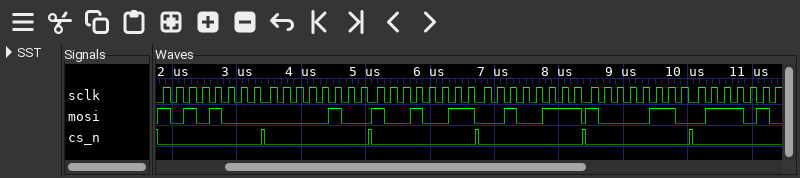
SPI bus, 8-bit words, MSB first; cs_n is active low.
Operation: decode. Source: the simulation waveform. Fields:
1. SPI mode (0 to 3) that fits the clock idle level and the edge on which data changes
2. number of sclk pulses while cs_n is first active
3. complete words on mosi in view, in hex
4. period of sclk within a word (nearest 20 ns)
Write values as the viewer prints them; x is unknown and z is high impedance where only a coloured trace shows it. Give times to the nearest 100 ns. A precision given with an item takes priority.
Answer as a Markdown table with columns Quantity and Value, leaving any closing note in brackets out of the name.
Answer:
| Quantity | Value |
|---|---|
| SPI mode (0 to 3) that fits the clock idle level and the edge on which data changes | 0 |
| number of sclk pulses while cs_n is first active | 8 |
| complete words on mosi in view, in hex | A8, 04, 93, 27, 86 |
| period of sclk within a word | 200 ns |
